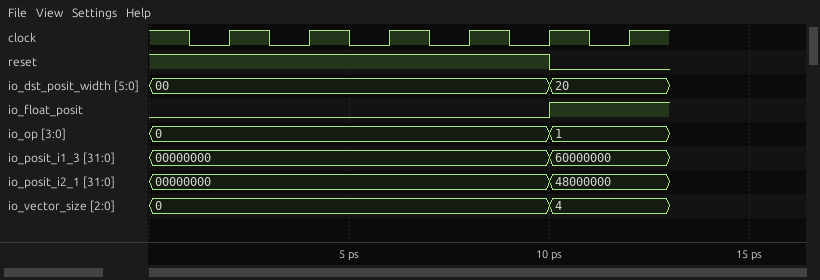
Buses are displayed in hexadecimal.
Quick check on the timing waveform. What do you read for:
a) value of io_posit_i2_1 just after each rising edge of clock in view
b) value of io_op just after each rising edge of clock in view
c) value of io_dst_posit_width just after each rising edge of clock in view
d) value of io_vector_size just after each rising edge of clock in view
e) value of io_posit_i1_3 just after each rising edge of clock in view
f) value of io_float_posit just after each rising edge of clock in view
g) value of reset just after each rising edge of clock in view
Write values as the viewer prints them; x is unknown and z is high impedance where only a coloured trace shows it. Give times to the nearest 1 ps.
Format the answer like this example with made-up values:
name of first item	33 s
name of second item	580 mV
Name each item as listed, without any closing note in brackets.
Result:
value of io_posit_i2_1 just after each rising edge of clock in view	00000000, 00000000, 00000000, 00000000, 48000000, 48000000
value of io_op just after each rising edge of clock in view	0, 0, 0, 0, 1, 1
value of io_dst_posit_width just after each rising edge of clock in view	00, 00, 00, 00, 20, 20
value of io_vector_size just after each rising edge of clock in view	0, 0, 0, 0, 4, 4
value of io_posit_i1_3 just after each rising edge of clock in view	00000000, 00000000, 00000000, 00000000, 60000000, 60000000
value of io_float_posit just after each rising edge of clock in view	0 0 0 0 1 1
value of reset just after each rising edge of clock in view	1 1 1 1 0 0
